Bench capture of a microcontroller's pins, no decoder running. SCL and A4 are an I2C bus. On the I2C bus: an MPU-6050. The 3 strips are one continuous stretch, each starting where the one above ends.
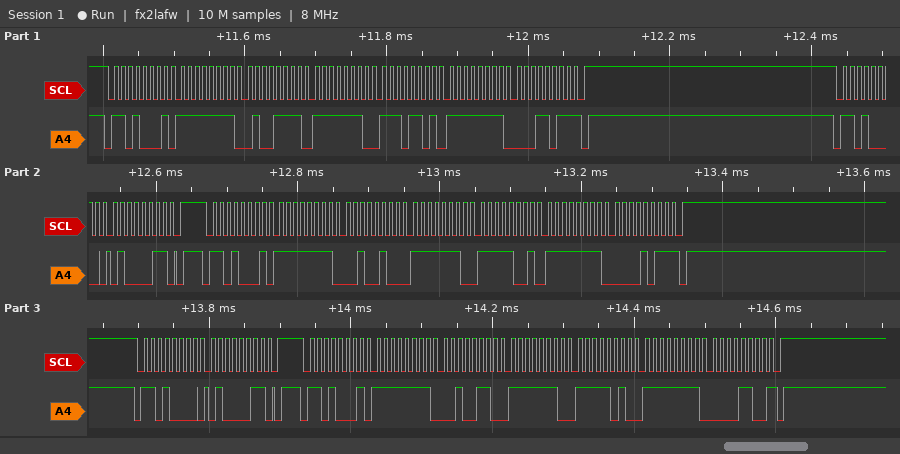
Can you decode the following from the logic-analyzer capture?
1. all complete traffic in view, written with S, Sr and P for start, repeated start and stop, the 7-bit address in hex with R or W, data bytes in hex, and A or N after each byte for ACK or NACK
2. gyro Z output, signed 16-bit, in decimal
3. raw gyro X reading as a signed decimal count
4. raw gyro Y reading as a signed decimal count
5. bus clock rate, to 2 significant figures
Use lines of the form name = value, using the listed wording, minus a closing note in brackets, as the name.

all complete traffic in view, written with S, Sr and P for start, repeated start and stop, the 7-bit address in hex with R or W, data bytes in hex, and A or N after each byte for ACK or NACK = S 68R A FF A 4F A FE A ED A FF A 1B N P S 68W A 43 A P S 68R A FF A 24 A FE A F9 A FF A 0B N P S 68W A 43 A P S 68R A FF A 26 A FE A FA A FF A 0C N P
gyro Z output, signed 16-bit, in decimal = -245
raw gyro X reading as a signed decimal count = -220
raw gyro Y reading as a signed decimal count = -263
bus clock rate, to 2 significant figures = 100 kHz
